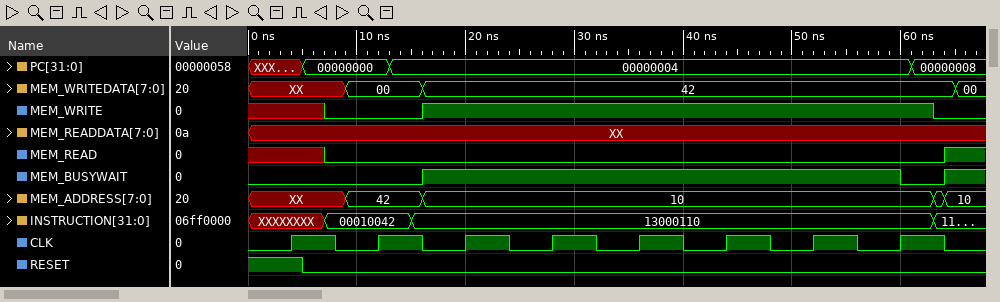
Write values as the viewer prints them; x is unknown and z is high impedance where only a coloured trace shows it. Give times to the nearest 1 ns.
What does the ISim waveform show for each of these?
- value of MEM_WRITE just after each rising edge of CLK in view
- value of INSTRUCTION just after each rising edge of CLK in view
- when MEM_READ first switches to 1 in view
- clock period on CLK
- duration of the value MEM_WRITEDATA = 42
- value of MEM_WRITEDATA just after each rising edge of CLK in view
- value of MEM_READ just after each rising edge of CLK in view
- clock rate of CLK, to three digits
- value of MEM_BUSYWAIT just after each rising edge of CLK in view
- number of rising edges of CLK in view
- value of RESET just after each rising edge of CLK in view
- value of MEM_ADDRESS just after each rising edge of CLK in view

x 0 1 1 1 1 1 1
XXXXXXXX, 00010042, 13000110, 13000110, 13000110, 13000110, 13000110, 13000110
64 ns
8 ns
49 ns
XX, 00, 42, 42, 42, 42, 42, 42
x 0 0 0 0 0 0 0
125 MHz
0 0 1 1 1 1 1 0
8
1 0 0 0 0 0 0 0
XX, 42, 10, 10, 10, 10, 10, 10
